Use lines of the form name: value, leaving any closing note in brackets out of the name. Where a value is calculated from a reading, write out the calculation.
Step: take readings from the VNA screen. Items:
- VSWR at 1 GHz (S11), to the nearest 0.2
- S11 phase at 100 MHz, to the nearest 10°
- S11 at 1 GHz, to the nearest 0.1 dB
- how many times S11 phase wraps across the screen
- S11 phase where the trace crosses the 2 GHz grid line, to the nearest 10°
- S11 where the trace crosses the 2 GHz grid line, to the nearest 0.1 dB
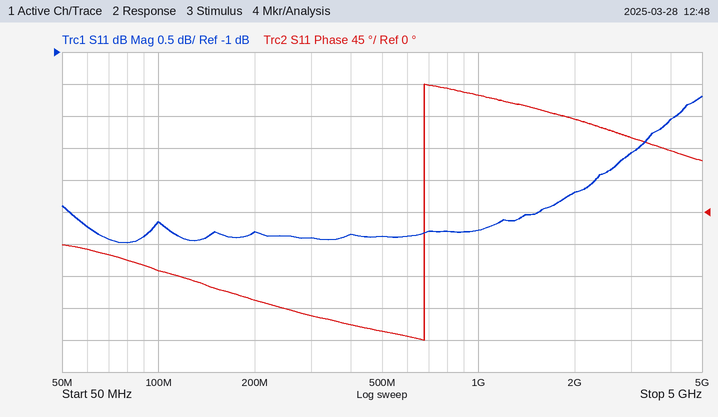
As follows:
VSWR at 1 GHz (S11), to the nearest 0.2: |Γ| = 10^(-3.8/20) = 0.6457; VSWR = (1 + 0.6457)/(1 − 0.6457) ≈ 4.6
S11 phase at 100 MHz, to the nearest 10°: -80°
S11 at 1 GHz, to the nearest 0.1 dB: -3.8 dB
how many times S11 phase wraps across the screen: 1
S11 phase where the trace crosses the 2 GHz grid line, to the nearest 10°: 130°
S11 where the trace crosses the 2 GHz grid line, to the nearest 0.1 dB: -3.2 dB
